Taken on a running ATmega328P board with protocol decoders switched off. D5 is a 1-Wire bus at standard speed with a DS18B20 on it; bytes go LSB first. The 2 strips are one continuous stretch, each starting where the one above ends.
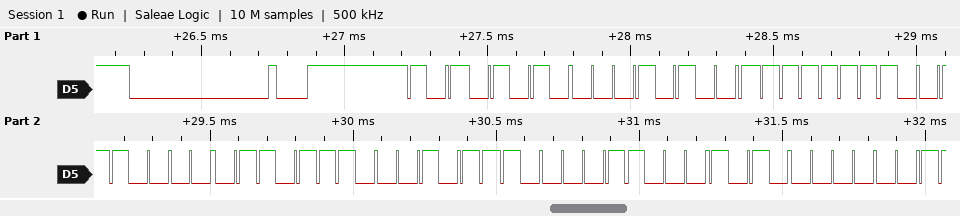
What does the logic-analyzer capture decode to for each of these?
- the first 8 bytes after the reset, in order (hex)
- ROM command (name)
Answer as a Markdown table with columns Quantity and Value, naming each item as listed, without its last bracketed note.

| Quantity | Value |
|---|---|
| the first 8 bytes after the reset, in order | 55 28 FF 0C 76 74 18 05 |
| ROM command | Match ROM |
